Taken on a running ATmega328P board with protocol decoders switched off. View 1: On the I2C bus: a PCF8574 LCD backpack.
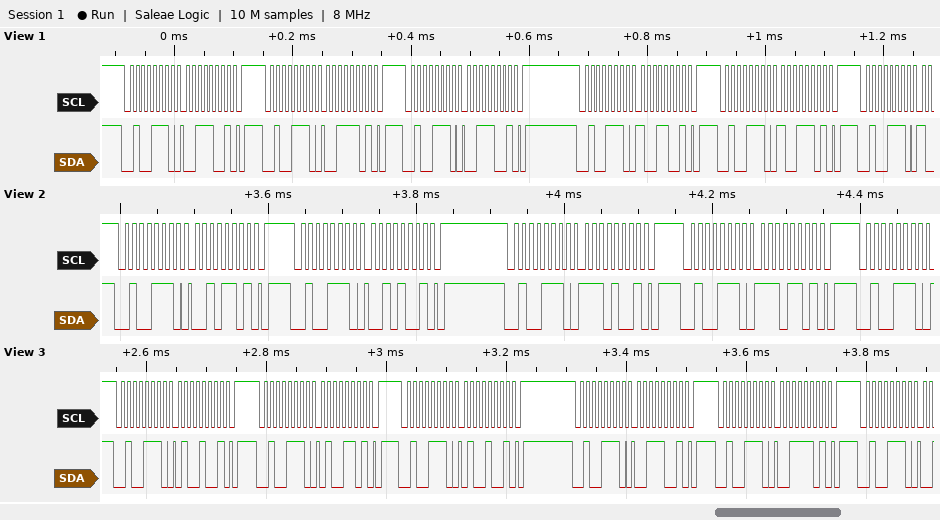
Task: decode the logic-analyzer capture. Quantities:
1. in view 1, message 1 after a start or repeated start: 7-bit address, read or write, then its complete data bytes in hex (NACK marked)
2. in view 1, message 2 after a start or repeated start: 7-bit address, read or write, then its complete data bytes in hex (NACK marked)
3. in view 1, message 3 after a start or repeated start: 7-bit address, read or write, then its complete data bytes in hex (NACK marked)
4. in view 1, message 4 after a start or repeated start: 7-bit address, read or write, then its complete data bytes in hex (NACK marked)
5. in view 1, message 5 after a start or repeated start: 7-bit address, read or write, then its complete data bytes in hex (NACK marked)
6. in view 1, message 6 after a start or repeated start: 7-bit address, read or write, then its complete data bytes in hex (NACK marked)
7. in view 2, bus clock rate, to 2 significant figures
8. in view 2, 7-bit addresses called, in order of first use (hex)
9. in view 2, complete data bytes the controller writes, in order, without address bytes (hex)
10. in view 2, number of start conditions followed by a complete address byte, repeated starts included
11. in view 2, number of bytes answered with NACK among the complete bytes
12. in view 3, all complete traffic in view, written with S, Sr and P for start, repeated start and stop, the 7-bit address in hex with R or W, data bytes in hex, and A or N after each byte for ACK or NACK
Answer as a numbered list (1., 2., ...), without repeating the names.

1. 0x27 write: 39
2. 0x27 write: 3D
3. 0x27 write: 39
4. 0x27 write: 99
5. 0x27 write: 9D
6. 0x27 write
7. 100 kHz
8. 0x27
9. 2D 29 E9 ED
10. 5
11. 0
12. S 27W A 49 A P S 27W A 4D A P S 27W A 49 A P S 27W A 39 A P S 27W A 3D A P S 27W A
